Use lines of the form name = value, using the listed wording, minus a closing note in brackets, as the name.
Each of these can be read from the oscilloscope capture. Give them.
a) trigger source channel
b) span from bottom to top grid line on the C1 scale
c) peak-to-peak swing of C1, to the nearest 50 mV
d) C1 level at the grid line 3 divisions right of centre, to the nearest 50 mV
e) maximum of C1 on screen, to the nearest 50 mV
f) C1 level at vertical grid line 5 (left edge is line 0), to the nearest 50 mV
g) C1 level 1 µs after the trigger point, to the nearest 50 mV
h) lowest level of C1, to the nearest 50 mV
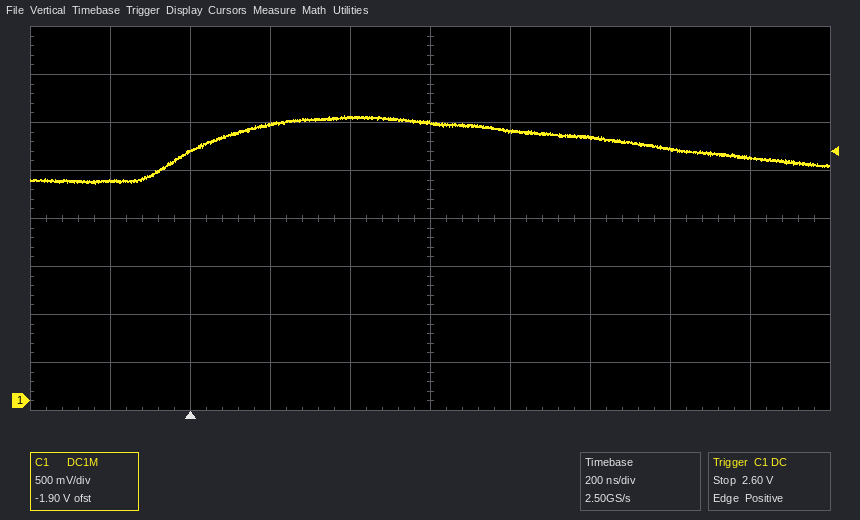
trigger source channel = C1
span from bottom to top grid line on the C1 scale = 4 V
peak-to-peak swing of C1, to the nearest 50 mV = 700 mV
C1 level at the grid line 3 divisions right of centre, to the nearest 50 mV = 2.60 V
maximum of C1 on screen, to the nearest 50 mV = 2.95 V
C1 level at vertical grid line 5 (left edge is line 0), to the nearest 50 mV = 2.90 V
C1 level 1 µs after the trigger point, to the nearest 50 mV = 2.75 V
lowest level of C1, to the nearest 50 mV = 2.25 V
